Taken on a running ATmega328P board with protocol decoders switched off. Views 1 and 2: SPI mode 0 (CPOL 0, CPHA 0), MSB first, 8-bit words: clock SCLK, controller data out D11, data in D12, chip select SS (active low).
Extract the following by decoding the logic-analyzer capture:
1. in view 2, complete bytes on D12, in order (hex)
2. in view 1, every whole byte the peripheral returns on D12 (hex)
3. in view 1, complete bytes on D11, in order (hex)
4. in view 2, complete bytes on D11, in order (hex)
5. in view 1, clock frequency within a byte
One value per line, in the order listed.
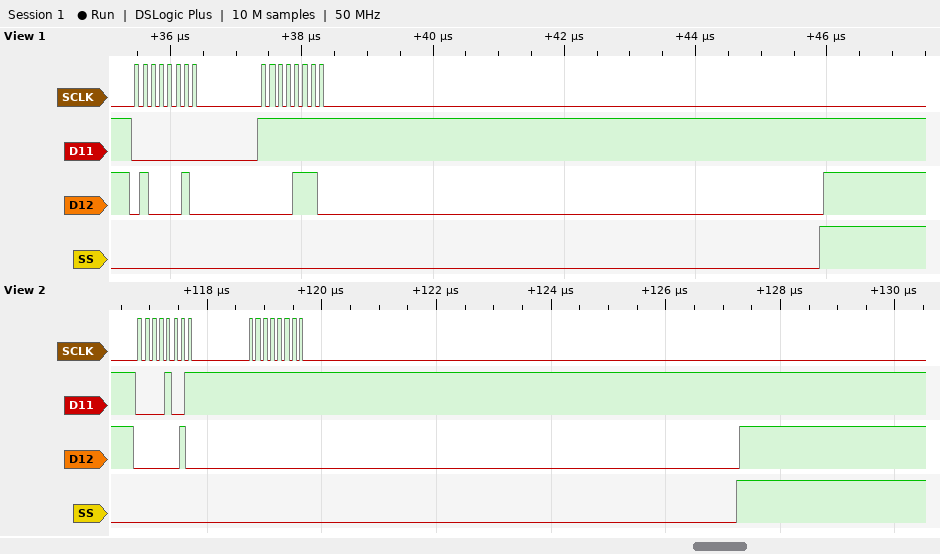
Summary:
0x02 0x00
42 0E
00 FF
0x09 0xFF
8 MHz
